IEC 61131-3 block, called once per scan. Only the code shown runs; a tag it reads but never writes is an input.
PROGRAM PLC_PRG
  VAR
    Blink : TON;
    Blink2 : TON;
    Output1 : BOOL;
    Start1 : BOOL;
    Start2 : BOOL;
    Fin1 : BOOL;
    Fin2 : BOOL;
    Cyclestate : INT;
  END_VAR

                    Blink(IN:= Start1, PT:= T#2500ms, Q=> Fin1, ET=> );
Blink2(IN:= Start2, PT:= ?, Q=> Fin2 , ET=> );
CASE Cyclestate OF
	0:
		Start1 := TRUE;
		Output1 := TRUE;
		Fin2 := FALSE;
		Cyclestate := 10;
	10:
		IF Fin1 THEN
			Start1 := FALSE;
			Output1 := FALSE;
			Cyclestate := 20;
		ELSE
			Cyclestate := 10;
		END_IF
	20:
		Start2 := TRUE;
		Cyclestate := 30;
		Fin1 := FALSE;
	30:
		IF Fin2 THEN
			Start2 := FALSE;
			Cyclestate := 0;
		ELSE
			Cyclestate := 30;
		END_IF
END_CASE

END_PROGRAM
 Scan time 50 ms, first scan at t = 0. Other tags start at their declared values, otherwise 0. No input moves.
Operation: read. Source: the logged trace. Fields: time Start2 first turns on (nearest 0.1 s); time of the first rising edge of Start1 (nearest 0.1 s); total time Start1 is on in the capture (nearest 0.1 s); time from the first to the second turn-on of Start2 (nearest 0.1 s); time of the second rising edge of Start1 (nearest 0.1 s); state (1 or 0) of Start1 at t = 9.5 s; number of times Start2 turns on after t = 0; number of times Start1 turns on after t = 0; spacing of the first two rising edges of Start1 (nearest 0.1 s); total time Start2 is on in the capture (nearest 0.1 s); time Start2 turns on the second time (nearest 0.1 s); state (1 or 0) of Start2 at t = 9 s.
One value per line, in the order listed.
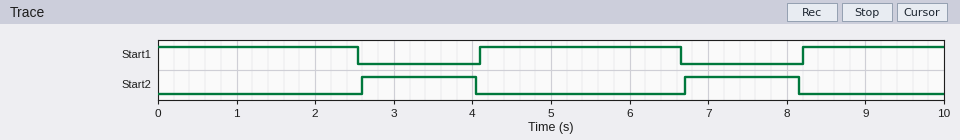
2.6 s
4.1 s
6.9 s
4.1 s
8.2 s
1
2
2
4.1 s
2.9 s
6.7 s
0
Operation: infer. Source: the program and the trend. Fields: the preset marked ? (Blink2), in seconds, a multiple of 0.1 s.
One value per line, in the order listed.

1.4 s
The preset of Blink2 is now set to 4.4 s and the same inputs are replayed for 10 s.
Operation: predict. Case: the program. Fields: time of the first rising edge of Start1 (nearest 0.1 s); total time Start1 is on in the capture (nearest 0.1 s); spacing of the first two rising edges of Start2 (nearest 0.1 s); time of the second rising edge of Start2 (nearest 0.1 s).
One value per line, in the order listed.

7.1 s
5.1 s
7.1 s
9.7 s
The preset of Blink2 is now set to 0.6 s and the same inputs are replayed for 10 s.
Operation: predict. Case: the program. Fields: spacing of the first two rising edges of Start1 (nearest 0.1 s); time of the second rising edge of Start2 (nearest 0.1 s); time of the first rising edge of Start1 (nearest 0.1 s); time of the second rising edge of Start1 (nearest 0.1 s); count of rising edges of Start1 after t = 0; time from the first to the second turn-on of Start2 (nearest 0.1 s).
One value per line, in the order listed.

3.3 s
5.9 s
3.3 s
6.6 s
3
3.3 s
